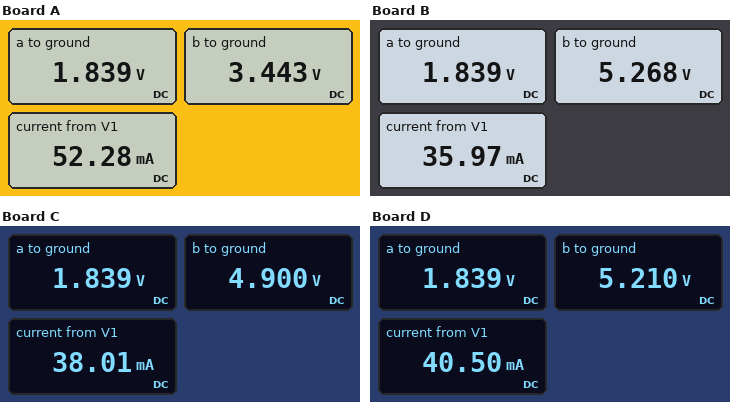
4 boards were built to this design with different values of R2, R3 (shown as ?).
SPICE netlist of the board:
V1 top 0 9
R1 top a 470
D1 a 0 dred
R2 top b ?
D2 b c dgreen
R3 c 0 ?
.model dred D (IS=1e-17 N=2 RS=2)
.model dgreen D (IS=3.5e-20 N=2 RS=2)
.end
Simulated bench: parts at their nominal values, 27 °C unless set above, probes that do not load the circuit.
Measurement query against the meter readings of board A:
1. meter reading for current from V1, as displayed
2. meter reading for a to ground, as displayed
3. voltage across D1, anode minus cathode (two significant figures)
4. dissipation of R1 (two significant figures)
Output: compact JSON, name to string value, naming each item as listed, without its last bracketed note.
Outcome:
{"meter reading for current from V1, as displayed": "52.28 mA", "meter reading for a to ground, as displayed": "1.839 V", "voltage across D1, anode minus cathode": "1.8 V", "dissipation of R1": "110 mW"}
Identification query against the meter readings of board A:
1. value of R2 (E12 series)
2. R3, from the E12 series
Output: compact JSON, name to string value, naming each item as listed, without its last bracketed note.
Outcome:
{"value of R2": "150 Ω", "R3, from the E12 series": "33 Ω"}
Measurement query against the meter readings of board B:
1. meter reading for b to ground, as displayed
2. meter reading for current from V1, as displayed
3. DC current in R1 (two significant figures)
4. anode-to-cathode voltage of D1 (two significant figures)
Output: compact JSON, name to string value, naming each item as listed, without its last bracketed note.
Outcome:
{"meter reading for b to ground, as displayed": "5.268 V", "meter reading for current from V1, as displayed": "35.97 mA", "DC current in R1": "15 mA", "anode-to-cathode voltage of D1": "1.8 V"}
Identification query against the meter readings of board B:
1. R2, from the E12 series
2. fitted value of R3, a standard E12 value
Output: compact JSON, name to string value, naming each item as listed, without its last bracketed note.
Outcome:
{"R2, from the E12 series": "180 Ω", "fitted value of R3, a standard E12 value": "150 Ω"}
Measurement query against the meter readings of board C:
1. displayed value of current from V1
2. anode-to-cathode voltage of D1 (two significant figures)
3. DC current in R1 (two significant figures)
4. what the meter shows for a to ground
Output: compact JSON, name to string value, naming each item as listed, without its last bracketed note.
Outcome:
{"displayed value of current from V1": "38.01 mA", "anode-to-cathode voltage of D1": "1.8 V", "DC current in R1": "15 mA", "what the meter shows for a to ground": "1.839 V"}
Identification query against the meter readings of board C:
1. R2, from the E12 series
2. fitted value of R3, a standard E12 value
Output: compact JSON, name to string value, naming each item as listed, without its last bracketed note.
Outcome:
{"R2, from the E12 series": "180 Ω", "fitted value of R3, a standard E12 value": "120 Ω"}
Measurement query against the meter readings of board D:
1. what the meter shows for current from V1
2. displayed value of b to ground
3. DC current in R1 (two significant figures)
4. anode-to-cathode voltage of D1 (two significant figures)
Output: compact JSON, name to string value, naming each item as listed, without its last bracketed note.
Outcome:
{"what the meter shows for current from V1": "40.50 mA", "displayed value of b to ground": "5.210 V", "DC current in R1": "15 mA", "anode-to-cathode voltage of D1": "1.8 V"}
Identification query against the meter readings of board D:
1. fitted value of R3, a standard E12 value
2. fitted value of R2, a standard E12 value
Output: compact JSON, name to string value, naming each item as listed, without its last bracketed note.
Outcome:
{"fitted value of R3, a standard E12 value": "120 Ω", "fitted value of R2, a standard E12 value": "150 Ω"}
